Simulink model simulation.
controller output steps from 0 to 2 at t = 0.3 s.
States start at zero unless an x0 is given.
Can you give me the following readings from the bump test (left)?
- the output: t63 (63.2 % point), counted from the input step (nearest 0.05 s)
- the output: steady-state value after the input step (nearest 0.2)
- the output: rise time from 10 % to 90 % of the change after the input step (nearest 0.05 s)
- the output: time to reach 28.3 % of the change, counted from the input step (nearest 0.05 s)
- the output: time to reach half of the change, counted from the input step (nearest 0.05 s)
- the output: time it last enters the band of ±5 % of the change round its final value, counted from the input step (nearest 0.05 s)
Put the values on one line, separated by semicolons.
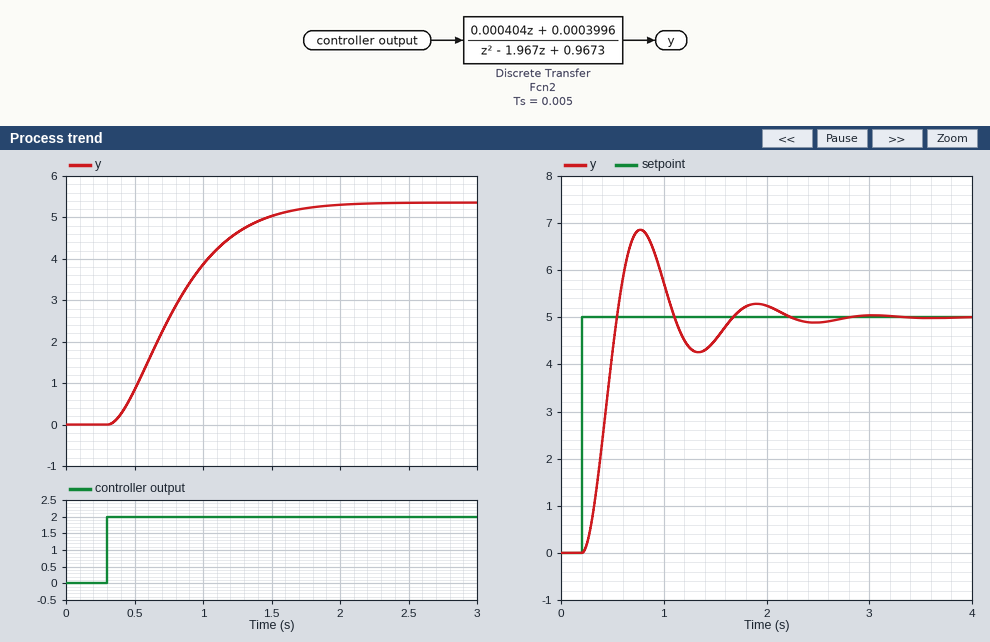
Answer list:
0.60 s; 5.4; 0.90 s; 0.30 s; 0.45 s; 1.25 s
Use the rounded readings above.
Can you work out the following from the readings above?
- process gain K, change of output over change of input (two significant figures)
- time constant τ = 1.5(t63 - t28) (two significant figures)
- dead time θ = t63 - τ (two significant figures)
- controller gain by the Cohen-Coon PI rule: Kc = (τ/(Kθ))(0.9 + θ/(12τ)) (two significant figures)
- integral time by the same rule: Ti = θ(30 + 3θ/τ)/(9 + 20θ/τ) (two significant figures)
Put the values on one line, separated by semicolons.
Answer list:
2.7; 0.45 s; 0.15 s; 1.0; 0.30 s
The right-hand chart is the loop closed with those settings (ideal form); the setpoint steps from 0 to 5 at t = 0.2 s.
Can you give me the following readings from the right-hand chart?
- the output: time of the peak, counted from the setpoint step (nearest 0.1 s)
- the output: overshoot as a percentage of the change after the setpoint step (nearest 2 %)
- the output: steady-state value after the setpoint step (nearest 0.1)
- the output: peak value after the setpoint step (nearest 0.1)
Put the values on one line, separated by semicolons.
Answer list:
0.6 s; 38 %; 5.0; 6.9
